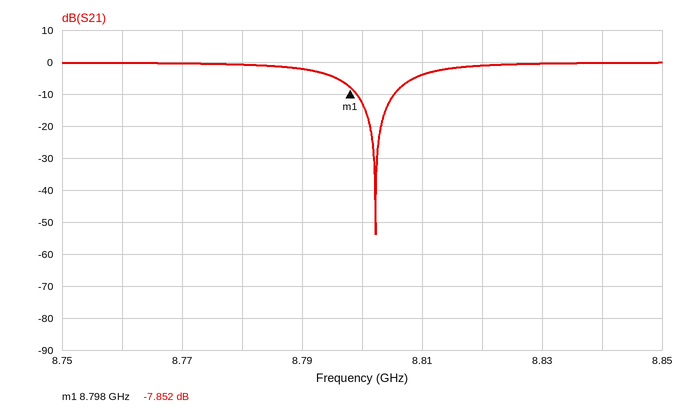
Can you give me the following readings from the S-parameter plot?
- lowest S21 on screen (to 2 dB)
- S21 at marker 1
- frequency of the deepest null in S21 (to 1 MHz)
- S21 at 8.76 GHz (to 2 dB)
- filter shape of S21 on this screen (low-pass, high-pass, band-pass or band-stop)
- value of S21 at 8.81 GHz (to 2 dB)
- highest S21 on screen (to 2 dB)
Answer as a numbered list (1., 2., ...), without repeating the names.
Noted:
1. -54 dB
2. -7.852 dB
3. 8.802 GHz
4. 0 dB
5. band-stop
6. -4 dB
7. 0 dB
